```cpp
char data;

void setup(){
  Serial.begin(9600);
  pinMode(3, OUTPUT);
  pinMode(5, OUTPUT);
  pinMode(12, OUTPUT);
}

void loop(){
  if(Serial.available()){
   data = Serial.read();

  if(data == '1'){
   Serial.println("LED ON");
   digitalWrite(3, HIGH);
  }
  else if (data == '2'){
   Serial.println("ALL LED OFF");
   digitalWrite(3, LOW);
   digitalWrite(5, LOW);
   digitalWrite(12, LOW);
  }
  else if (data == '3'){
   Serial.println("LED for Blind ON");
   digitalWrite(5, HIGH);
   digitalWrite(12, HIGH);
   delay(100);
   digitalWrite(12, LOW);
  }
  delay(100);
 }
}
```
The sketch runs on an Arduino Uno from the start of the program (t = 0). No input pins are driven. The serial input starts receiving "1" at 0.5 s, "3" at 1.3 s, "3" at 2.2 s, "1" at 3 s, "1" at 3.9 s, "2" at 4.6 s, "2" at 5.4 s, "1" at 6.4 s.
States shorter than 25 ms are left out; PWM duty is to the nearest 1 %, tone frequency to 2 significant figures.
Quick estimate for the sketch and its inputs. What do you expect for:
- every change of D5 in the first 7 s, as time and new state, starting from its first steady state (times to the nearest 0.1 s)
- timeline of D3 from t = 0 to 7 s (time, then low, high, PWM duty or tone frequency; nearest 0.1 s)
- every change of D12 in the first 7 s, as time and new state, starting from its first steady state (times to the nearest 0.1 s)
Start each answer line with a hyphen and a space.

- 0 s low; 1.3 s high; 4.6 s low
- 0 s low; 0.5 s high; 4.6 s low; 6.4 s high
- 0 s low; 1.3 s high; 1.4 s low; 2.2 s high; 2.3 s low
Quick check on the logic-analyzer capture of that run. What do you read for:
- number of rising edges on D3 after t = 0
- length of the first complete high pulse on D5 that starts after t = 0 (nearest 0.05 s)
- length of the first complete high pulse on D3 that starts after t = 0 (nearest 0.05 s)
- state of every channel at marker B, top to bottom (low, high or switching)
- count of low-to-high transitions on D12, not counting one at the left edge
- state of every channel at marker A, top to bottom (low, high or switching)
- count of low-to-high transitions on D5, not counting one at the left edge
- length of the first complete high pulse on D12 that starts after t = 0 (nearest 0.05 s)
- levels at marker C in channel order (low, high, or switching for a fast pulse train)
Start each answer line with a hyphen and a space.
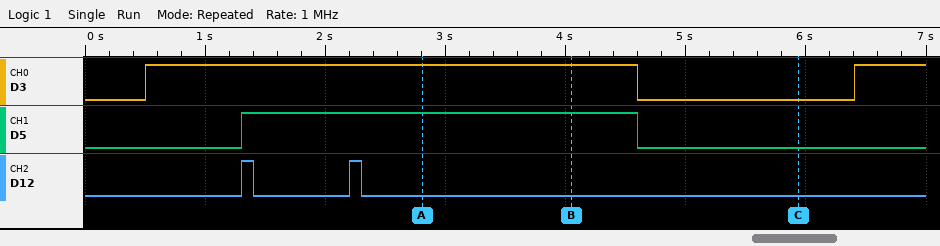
- 2
- 3.30 s
- 4.10 s
- D3 high, D5 high, D12 low
- 2
- D3 high, D5 high, D12 low
- 1
- 0.10 s
- D3 low, D5 low, D12 low
